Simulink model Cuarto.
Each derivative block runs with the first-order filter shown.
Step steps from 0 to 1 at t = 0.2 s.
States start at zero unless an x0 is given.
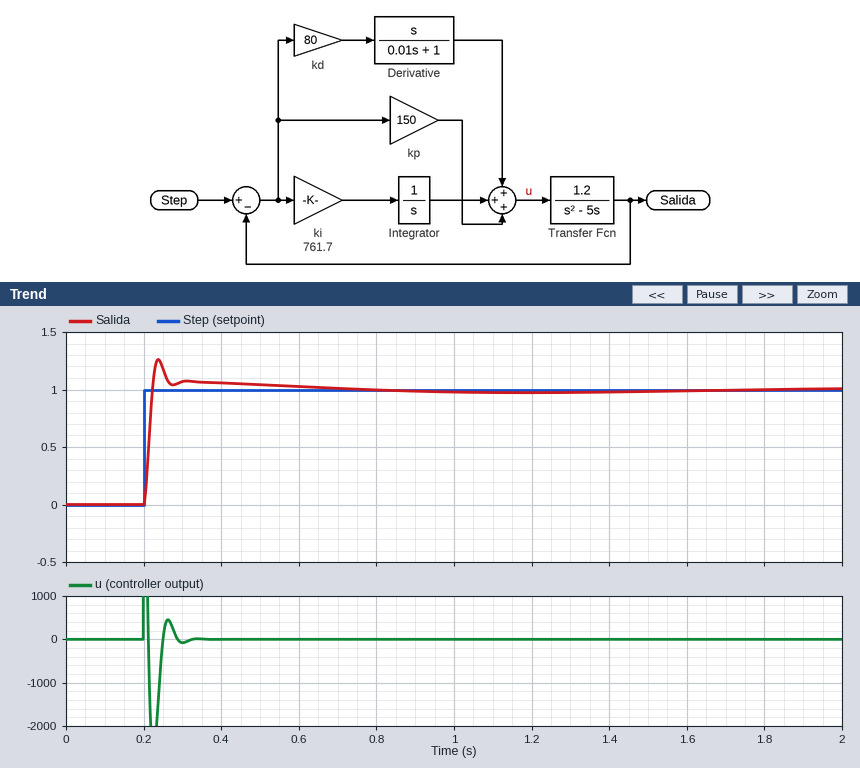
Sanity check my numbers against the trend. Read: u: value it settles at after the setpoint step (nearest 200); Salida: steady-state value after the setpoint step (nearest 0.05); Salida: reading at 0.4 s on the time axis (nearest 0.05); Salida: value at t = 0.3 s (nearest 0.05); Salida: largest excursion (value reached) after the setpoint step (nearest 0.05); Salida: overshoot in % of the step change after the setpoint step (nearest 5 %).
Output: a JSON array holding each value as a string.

["0", "1.00", "1.05", "1.05", "1.25", "25 %"]
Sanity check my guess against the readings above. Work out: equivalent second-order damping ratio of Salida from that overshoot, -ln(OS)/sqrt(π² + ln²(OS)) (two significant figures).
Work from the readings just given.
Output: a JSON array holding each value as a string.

["0.40"]
